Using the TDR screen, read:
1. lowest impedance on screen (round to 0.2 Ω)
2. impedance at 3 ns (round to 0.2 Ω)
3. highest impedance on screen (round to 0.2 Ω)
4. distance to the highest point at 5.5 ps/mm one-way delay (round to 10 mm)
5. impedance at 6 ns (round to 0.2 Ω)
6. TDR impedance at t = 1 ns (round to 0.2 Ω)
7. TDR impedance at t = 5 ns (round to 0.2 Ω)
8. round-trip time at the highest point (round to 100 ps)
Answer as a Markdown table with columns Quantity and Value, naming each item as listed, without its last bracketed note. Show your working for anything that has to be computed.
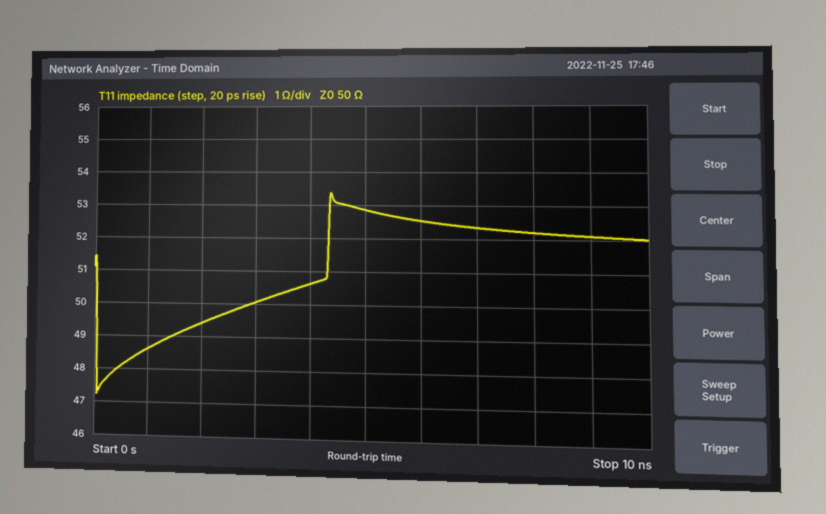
| Quantity | Value |
|---|---|
| lowest impedance on screen | 47.2 Ω |
| impedance at 3 ns | 50.0 Ω |
| highest impedance on screen | 53.4 Ω |
| distance to the highest point at 5.5 ps/mm one-way delay | 4.4 ns / 2 / 5.5 ps/mm ≈ 400 mm |
| impedance at 6 ns | 52.6 Ω |
| TDR impedance at t = 1 ns | 48.6 Ω |
| TDR impedance at t = 5 ns | 52.8 Ω |
| round-trip time at the highest point | 4.4 ns |
